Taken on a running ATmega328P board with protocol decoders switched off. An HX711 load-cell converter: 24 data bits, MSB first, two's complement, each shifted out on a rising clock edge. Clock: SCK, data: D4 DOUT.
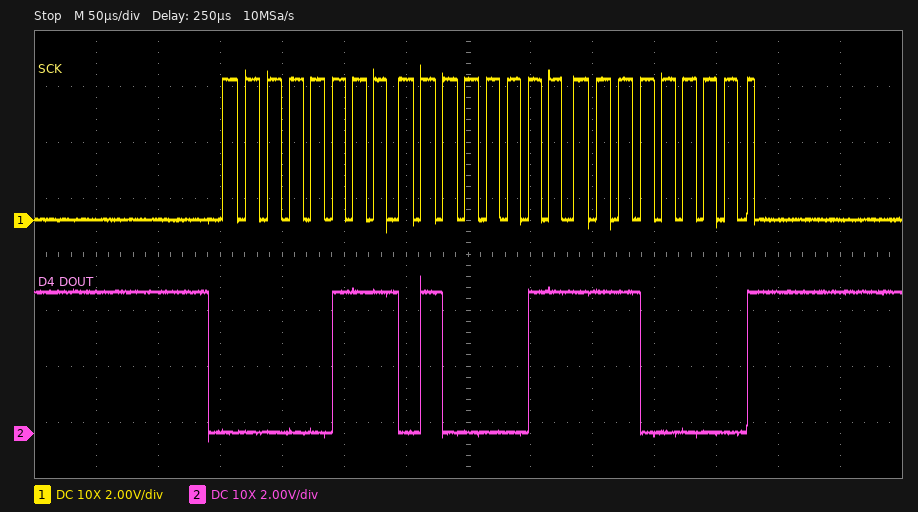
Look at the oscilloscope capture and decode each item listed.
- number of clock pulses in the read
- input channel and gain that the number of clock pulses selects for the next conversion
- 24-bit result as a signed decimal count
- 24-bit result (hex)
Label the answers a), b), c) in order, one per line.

a) 25
b) channel A, gain 128
c) 476128
d) 0x0743E0
